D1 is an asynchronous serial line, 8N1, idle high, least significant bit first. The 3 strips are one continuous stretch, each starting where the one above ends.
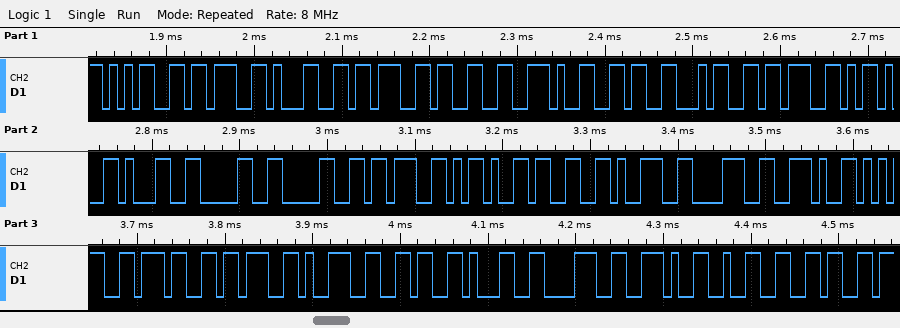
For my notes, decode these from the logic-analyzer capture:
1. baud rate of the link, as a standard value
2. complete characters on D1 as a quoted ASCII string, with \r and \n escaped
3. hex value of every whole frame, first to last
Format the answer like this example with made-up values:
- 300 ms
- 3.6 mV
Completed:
- 115200 baud
- "5;1;3.64;-100;-398.57;9618.26"
- 35 3B 31 3B 33 2E 36 34 3B 2D 31 30 30 3B 2D 33 39 38 2E 35 37 3B 39 36 31 38 2E 32 36
